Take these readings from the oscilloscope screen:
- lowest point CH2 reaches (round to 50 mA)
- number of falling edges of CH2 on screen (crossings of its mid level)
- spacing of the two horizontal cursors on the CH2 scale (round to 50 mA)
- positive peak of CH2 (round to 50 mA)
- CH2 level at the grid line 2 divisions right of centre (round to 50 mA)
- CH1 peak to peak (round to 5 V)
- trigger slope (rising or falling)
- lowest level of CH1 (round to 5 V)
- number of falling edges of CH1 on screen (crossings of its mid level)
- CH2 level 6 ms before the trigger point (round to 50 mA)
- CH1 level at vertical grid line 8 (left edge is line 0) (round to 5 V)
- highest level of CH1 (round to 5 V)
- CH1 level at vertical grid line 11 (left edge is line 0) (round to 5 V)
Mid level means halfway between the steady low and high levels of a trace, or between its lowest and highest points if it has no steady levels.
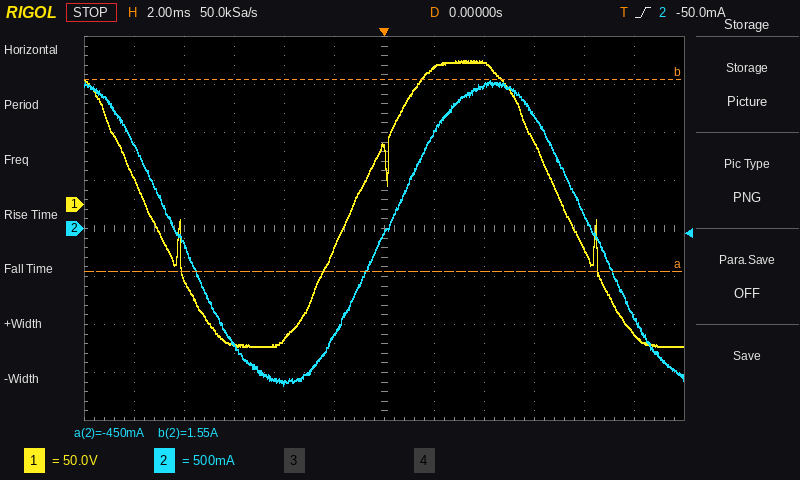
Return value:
-1.65 A
2
2.00 A
1.55 A
1.50 A
300 V
rising
-150 V
2
-1.20 A
150 V
150 V
-135 V
